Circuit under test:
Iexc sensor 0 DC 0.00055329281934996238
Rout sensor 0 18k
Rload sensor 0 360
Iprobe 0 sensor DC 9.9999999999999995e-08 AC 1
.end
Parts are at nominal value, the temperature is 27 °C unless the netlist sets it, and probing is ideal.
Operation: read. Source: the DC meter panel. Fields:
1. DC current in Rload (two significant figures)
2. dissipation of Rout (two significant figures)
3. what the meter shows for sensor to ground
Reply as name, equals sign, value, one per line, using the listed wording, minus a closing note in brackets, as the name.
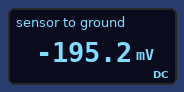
DC current in Rload = 540 µA
dissipation of Rout = 2.1 µW
what the meter shows for sensor to ground = -195.2 mV
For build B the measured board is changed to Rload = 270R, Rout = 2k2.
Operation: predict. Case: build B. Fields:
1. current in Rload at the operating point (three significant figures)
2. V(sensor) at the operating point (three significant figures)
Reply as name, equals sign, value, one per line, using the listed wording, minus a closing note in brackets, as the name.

current in Rload at the operating point = 493 µA
V(sensor) at the operating point = -133 mV
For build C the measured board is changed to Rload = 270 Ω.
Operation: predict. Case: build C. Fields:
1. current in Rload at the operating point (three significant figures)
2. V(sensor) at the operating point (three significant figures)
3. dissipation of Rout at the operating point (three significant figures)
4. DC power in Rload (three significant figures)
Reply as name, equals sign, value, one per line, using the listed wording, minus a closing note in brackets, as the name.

current in Rload at the operating point = 545 µA
V(sensor) at the operating point = -147 mV
dissipation of Rout at the operating point = 1.20 µW
DC power in Rload = 80.2 µW
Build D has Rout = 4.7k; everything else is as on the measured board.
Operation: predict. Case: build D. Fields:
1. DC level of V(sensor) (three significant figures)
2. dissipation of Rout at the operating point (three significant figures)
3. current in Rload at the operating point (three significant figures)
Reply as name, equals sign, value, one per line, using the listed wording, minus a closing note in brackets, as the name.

DC level of V(sensor) = -185 mV
dissipation of Rout at the operating point = 7.28 µW
current in Rload at the operating point = 514 µA
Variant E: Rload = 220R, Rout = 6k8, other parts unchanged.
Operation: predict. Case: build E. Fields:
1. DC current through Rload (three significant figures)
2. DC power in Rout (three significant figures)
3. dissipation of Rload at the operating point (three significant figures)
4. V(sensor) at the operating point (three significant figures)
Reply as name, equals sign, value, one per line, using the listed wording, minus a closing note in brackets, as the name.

DC current through Rload = 536 µA
DC power in Rout = 2.04 µW
dissipation of Rload at the operating point = 63.2 µW
V(sensor) at the operating point = -118 mV
